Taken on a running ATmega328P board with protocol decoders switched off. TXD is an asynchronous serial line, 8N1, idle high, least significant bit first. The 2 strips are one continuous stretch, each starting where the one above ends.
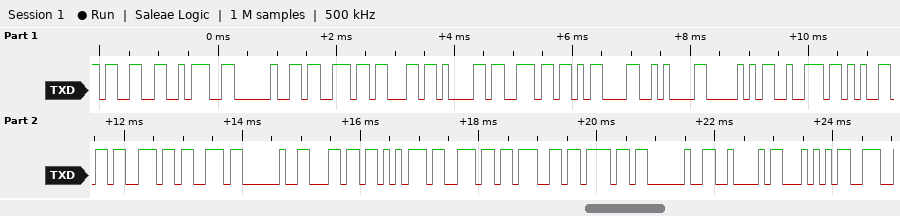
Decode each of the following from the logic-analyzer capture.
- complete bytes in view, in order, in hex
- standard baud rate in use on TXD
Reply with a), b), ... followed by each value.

a) 33 3A 20 73 63 61 6E 0D 0A 50 72 65 73 73 20 6C 75 6E 67 6F 20 42 54
b) 9600 baud
